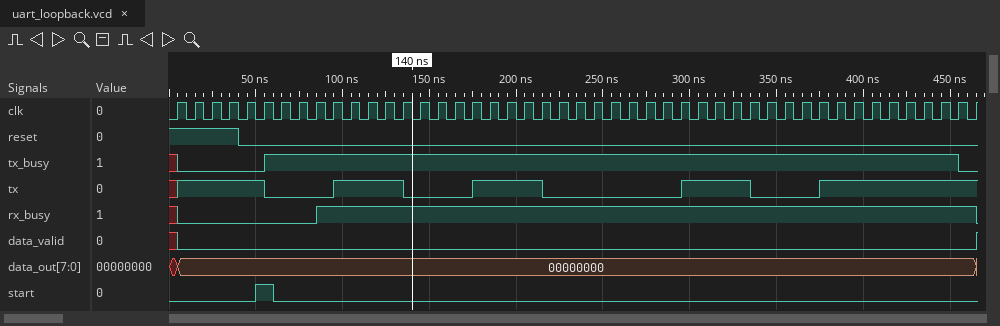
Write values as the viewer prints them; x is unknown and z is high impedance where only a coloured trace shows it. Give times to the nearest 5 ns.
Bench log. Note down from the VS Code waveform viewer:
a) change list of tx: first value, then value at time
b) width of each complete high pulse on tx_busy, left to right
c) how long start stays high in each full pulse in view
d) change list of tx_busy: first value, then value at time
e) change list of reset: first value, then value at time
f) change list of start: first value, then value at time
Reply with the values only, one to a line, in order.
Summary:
x, 1 at 5 ns, 0 at 55 ns, 1 at 95 ns, 0 at 135 ns, 1 at 175 ns, 0 at 215 ns, 1 at 295 ns, 0 at 335 ns, 1 at 375 ns
400 ns
10 ns
x, 0 at 5 ns, 1 at 55 ns, 0 at 455 ns
1, 0 at 40 ns
0, 1 at 50 ns, 0 at 60 ns
